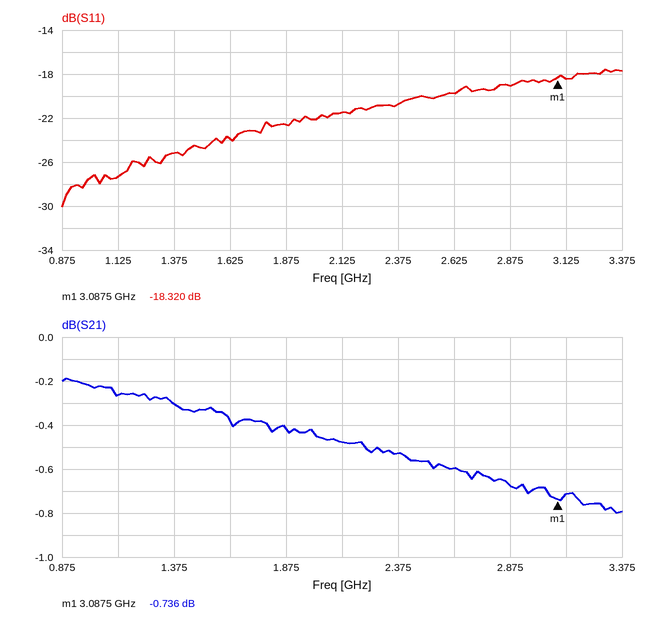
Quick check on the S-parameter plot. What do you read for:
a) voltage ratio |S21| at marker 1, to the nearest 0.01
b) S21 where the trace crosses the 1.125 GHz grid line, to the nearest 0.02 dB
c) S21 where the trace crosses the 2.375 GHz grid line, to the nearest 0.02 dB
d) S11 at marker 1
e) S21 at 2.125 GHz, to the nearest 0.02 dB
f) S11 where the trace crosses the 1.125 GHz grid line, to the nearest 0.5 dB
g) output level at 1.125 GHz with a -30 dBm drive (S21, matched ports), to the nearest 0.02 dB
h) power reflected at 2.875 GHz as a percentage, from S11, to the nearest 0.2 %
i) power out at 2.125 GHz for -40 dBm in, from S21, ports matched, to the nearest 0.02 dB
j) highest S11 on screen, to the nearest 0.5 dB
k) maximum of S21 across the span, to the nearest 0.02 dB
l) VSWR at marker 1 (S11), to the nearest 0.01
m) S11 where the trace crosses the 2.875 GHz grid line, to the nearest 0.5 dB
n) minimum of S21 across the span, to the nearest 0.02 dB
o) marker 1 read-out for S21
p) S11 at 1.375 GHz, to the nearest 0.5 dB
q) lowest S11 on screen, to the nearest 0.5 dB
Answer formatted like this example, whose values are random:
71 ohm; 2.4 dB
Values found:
0.92; -0.26 dB; -0.52 dB; -18.320 dB; -0.48 dB; -27.5 dB; -30.26 dBm; 1.2 %; -40.48 dBm; -17.5 dB; -0.18 dB; 1.28; -19.0 dB; -0.80 dB; -0.736 dB; -25.0 dB; -30.0 dB
